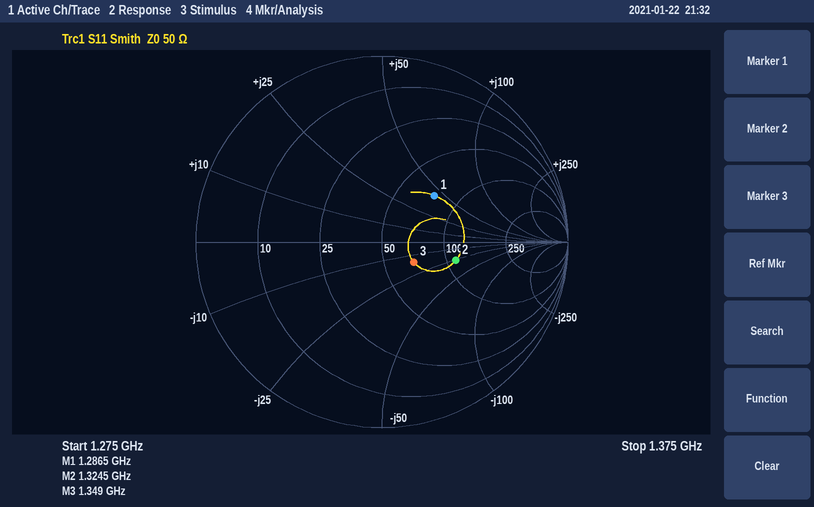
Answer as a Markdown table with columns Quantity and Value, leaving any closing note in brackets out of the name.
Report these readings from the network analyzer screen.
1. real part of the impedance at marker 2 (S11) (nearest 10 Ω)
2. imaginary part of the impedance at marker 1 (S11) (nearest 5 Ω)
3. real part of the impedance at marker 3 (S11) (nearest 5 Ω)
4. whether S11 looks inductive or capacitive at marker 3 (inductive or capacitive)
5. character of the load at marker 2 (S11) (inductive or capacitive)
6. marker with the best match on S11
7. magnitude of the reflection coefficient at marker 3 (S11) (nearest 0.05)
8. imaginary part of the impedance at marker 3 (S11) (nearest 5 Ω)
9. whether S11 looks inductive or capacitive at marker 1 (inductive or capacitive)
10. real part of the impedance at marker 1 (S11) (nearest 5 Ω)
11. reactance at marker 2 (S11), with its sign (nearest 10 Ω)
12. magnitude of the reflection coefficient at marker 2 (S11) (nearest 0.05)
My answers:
| Quantity | Value |
|---|---|
| real part of the impedance at marker 2 (S11) | 110 Ω |
| imaginary part of the impedance at marker 1 (S11) | +45 Ω |
| real part of the impedance at marker 3 (S11) | 70 Ω |
| whether S11 looks inductive or capacitive at marker 3 | capacitive |
| character of the load at marker 2 (S11) | capacitive |
| marker with the best match on S11 | marker 3 |
| magnitude of the reflection coefficient at marker 3 (S11) | 0.20 |
| imaginary part of the impedance at marker 3 (S11) | -15 Ω |
| whether S11 looks inductive or capacitive at marker 1 | inductive |
| real part of the impedance at marker 1 (S11) | 75 Ω |
| reactance at marker 2 (S11), with its sign | -30 Ω |
| magnitude of the reflection coefficient at marker 2 (S11) | 0.40 |
